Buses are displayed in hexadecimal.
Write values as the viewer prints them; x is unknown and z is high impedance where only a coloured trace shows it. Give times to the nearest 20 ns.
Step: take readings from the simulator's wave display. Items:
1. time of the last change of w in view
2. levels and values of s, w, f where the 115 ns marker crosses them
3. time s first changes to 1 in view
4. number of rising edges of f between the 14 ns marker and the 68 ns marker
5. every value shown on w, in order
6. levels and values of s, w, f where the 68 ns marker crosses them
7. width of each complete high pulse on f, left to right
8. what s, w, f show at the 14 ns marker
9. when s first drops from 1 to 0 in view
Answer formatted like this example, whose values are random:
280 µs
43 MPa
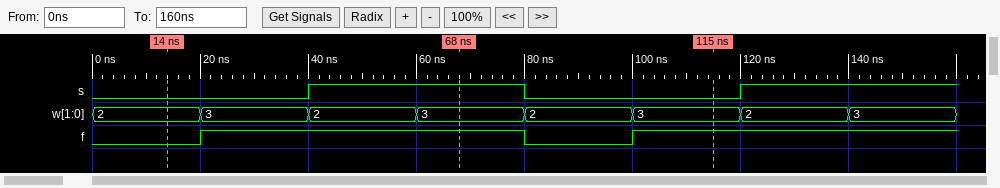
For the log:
140 ns
s=0, w=3, f=1
40 ns
1
2, 3, 2, 3, 2, 3, 2, 3
s=1, w=3, f=1
60 ns
s=0, w=2, f=0
80 ns
